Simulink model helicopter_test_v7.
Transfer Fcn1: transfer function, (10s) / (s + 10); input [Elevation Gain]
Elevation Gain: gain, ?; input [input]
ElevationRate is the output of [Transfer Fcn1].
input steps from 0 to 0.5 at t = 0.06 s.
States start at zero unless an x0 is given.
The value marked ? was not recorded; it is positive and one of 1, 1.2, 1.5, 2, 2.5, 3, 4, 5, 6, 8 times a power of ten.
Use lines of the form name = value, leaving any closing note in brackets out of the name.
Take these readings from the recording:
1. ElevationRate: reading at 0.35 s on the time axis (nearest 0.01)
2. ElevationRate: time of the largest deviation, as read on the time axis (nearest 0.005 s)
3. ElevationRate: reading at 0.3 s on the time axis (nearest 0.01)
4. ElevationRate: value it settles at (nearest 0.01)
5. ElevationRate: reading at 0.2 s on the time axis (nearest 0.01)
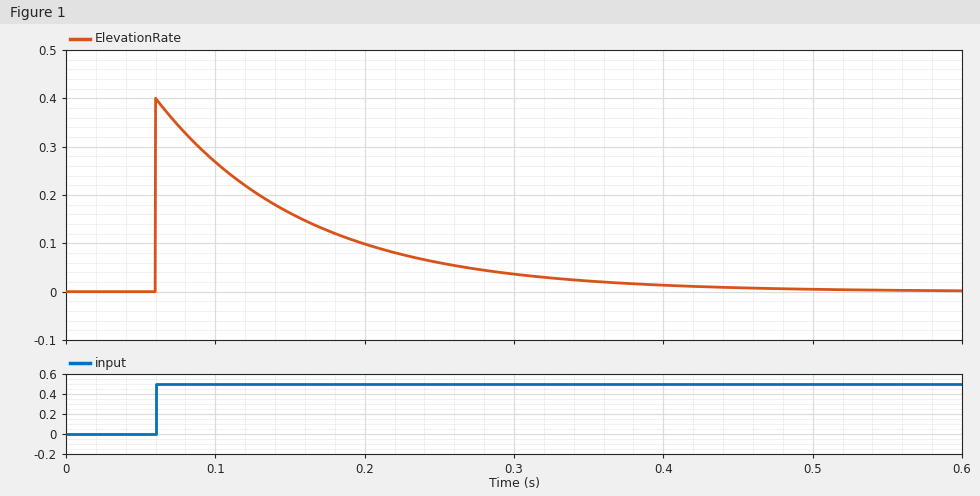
ElevationRate: reading at 0.35 s on the time axis = 0.02
ElevationRate: time of the largest deviation, as read on the time axis = 0.060 s
ElevationRate: reading at 0.3 s on the time axis = 0.04
ElevationRate: value it settles at = 0.00
ElevationRate: reading at 0.2 s on the time axis = 0.10
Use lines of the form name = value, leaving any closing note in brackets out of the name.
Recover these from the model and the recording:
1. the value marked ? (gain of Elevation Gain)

the value marked ? = 0.08
